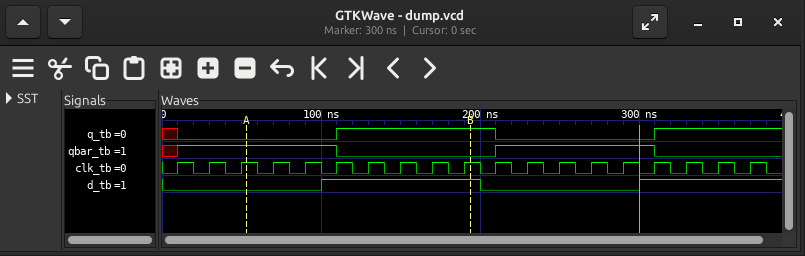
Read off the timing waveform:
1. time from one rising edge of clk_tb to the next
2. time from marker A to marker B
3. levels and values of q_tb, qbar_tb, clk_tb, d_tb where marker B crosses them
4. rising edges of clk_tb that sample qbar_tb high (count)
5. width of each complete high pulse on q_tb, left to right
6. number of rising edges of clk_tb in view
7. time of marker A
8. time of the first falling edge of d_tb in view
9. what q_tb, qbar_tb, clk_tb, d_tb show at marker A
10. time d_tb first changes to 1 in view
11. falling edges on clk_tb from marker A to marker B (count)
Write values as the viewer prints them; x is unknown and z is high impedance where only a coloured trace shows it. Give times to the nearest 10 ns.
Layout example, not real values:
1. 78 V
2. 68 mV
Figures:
1. 20 ns
2. 140 ns
3. q_tb=1, qbar_tb=0, clk_tb=1, d_tb=1
4. 10
5. 100 ns
6. 19
7. 50 ns
8. 200 ns
9. q_tb=0, qbar_tb=1, clk_tb=1, d_tb=0
10. 100 ns
11. 7
